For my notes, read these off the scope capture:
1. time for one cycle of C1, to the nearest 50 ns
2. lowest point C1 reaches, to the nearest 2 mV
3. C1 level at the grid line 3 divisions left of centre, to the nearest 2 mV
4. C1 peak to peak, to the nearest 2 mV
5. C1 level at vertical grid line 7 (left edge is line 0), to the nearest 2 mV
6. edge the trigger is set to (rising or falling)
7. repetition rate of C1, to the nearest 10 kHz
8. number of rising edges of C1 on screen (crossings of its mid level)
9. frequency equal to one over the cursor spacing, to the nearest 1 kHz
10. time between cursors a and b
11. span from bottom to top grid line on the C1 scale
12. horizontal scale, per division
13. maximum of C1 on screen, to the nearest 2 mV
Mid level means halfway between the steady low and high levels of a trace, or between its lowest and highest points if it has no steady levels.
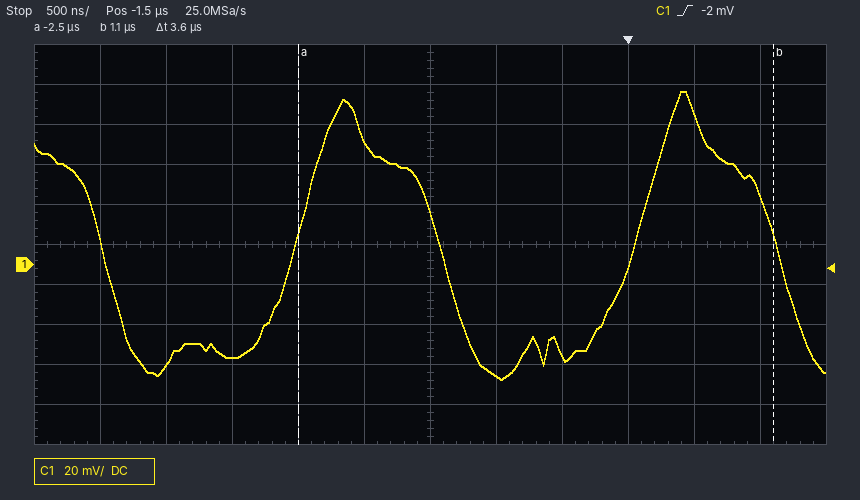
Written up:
2.55 µs
-58 mV
-46 mV
144 mV
-56 mV
rising
390 kHz
2
278 kHz
3.6 µs
200 mV
500 ns
86 mV
